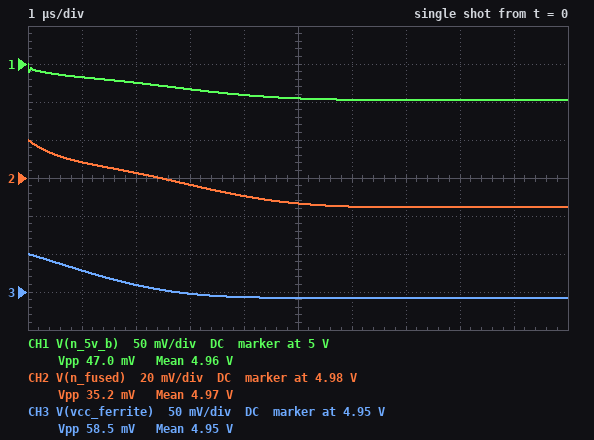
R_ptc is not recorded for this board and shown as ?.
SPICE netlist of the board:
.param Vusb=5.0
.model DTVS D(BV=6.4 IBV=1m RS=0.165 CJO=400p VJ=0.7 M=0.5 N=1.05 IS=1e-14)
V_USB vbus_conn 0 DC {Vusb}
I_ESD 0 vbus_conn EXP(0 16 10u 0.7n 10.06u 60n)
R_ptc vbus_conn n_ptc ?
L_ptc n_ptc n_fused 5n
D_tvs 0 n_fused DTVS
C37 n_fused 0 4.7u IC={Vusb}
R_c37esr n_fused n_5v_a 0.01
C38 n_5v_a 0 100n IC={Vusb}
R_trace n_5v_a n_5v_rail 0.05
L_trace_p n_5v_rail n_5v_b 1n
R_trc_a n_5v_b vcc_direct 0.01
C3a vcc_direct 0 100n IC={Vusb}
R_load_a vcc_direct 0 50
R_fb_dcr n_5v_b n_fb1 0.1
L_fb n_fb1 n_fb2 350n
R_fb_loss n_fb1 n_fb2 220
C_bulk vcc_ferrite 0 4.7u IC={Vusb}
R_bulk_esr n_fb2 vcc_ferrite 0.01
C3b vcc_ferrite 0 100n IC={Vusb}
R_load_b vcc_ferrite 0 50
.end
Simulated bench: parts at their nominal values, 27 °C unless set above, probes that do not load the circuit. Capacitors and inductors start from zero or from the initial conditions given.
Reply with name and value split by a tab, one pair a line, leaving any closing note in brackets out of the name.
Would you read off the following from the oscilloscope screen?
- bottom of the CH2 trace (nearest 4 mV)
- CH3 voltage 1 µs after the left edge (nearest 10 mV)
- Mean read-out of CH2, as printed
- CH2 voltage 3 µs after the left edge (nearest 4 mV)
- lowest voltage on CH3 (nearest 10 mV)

bottom of the CH2 trace	4.964 V
CH3 voltage 1 µs after the left edge	4.98 V
Mean read-out of CH2, as printed	4.97 V
CH2 voltage 3 µs after the left edge	4.976 V
lowest voltage on CH3	4.94 V
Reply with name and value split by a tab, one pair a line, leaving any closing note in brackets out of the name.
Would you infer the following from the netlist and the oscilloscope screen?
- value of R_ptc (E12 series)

value of R_ptc	0.18 Ω
